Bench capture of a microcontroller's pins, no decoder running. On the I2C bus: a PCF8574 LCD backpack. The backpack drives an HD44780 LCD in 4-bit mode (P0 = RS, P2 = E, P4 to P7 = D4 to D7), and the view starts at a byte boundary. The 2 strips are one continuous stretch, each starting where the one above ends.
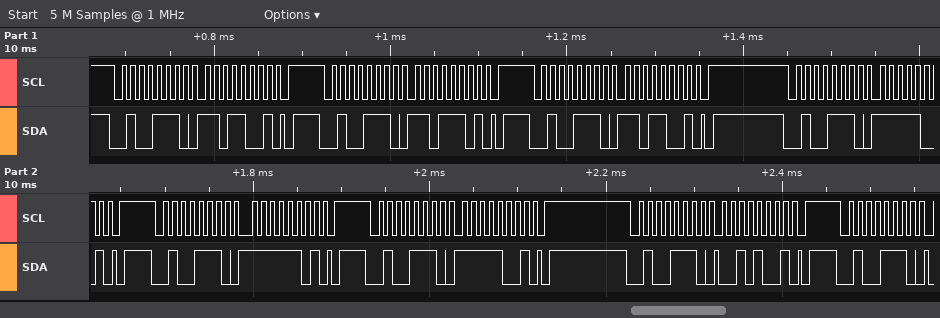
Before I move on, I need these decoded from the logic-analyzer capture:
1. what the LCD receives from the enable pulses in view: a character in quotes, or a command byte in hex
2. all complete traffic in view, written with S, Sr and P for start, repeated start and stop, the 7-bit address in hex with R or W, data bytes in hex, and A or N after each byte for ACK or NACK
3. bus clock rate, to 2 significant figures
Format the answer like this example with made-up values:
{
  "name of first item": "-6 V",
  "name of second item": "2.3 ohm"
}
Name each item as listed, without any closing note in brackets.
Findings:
{
  "what the LCD receives from the enable pulses in view: a character in quotes, or a command byte in hex": "data 0xDF",
  "all complete traffic in view, written with S, Sr and P for start, repeated start and stop, the 7-bit address in hex with R or W, data bytes in hex, and A or N after each byte for ACK or NACK": "S 27W A D9 A P S 27W A DD A P S 27W A D9 A P S 27W A F9 A P S 27W A FD A P S 27W A F9 A P S 27W A 29 A P S 27W A",
  "bus clock rate, to 2 significant figures": "100 kHz"
}
